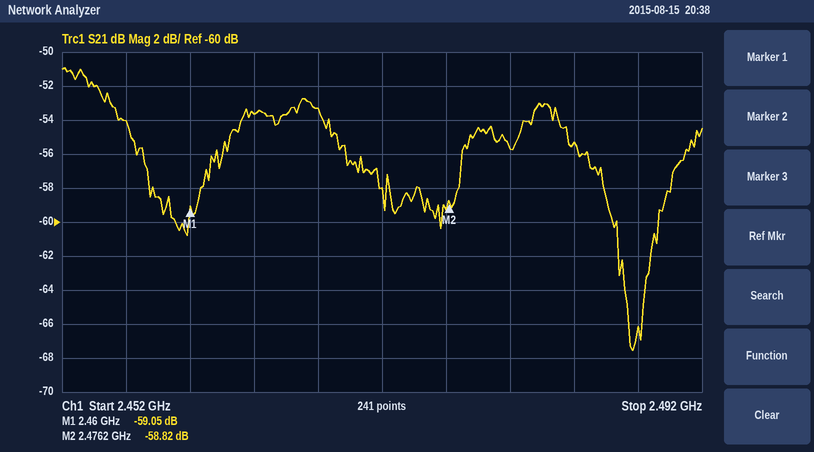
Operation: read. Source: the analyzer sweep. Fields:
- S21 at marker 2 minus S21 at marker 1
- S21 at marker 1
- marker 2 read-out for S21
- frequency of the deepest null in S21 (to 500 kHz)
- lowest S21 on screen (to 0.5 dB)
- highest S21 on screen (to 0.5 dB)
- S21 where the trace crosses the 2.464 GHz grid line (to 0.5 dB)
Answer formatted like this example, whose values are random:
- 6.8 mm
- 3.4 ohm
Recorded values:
- 0.23 dB
- -59.05 dB
- -58.82 dB
- 2.4875 GHz
- -67.5 dB
- -51.0 dB
- -53.5 dB
